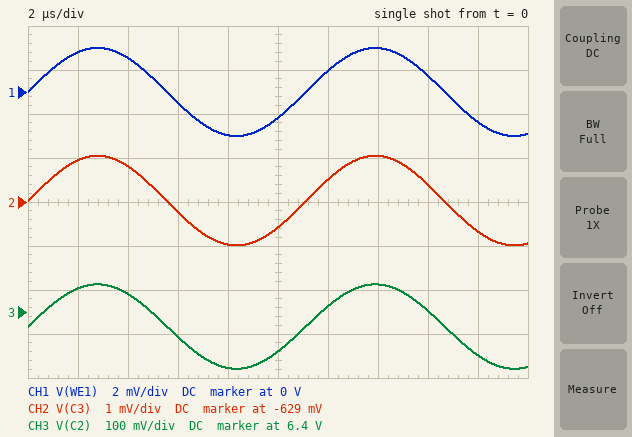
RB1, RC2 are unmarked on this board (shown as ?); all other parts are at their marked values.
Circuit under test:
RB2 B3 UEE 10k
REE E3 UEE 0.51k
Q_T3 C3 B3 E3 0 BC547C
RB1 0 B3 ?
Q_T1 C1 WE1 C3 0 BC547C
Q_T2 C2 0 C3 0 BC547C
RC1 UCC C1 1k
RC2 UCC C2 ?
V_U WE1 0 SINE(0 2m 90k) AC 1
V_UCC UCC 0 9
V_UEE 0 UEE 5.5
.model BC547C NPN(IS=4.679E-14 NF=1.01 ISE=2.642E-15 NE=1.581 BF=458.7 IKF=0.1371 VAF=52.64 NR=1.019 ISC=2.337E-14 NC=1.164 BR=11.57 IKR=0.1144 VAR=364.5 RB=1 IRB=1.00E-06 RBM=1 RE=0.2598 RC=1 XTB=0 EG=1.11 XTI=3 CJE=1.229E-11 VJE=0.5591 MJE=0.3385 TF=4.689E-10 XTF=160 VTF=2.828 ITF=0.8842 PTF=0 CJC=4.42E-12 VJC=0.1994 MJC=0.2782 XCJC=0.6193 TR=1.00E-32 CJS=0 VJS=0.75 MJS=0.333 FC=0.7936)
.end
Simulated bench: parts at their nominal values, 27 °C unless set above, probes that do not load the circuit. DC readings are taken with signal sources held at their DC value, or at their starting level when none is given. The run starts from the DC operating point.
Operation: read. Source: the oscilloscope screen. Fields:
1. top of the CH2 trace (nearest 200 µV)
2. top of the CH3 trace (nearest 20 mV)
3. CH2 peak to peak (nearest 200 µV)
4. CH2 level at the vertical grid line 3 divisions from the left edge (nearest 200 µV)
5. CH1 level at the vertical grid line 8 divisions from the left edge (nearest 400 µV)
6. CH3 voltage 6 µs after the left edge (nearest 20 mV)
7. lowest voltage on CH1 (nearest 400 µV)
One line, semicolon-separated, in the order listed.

-628.0 mV; 6.46 V; 2.0 mV; -629.2 mV; 800 µV; 6.34 V; -2.0 mV
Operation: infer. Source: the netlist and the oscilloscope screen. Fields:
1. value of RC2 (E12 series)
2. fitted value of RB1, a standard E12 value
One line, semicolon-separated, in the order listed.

1.8 kΩ; 15 kΩ
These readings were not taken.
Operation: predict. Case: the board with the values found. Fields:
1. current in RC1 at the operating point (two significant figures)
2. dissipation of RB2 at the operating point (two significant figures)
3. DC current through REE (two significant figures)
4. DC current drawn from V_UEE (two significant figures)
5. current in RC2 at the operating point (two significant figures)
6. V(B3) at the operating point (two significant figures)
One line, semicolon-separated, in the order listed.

1.5 mA; 470 µW; 3.0 mA; 3.2 mA; 1.5 mA; -3.3 V
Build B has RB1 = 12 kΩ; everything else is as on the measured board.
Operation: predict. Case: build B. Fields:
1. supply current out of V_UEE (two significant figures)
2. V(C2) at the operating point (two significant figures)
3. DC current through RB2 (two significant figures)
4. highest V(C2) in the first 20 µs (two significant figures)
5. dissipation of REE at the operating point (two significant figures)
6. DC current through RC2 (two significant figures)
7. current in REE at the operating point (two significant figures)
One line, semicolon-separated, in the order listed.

3.8 mA; 5.9 V; 250 µA; 6.0 V; 6.4 mW; 1.7 mA; 3.5 mA
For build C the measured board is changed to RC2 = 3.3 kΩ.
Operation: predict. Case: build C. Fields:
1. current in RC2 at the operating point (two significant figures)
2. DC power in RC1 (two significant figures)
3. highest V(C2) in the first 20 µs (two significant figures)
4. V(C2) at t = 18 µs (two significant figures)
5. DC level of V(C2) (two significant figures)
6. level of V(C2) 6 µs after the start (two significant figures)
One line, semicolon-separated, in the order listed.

1.4 mA; 2.3 mW; 4.4 V; 4.1 V; 4.3 V; 4.2 V
